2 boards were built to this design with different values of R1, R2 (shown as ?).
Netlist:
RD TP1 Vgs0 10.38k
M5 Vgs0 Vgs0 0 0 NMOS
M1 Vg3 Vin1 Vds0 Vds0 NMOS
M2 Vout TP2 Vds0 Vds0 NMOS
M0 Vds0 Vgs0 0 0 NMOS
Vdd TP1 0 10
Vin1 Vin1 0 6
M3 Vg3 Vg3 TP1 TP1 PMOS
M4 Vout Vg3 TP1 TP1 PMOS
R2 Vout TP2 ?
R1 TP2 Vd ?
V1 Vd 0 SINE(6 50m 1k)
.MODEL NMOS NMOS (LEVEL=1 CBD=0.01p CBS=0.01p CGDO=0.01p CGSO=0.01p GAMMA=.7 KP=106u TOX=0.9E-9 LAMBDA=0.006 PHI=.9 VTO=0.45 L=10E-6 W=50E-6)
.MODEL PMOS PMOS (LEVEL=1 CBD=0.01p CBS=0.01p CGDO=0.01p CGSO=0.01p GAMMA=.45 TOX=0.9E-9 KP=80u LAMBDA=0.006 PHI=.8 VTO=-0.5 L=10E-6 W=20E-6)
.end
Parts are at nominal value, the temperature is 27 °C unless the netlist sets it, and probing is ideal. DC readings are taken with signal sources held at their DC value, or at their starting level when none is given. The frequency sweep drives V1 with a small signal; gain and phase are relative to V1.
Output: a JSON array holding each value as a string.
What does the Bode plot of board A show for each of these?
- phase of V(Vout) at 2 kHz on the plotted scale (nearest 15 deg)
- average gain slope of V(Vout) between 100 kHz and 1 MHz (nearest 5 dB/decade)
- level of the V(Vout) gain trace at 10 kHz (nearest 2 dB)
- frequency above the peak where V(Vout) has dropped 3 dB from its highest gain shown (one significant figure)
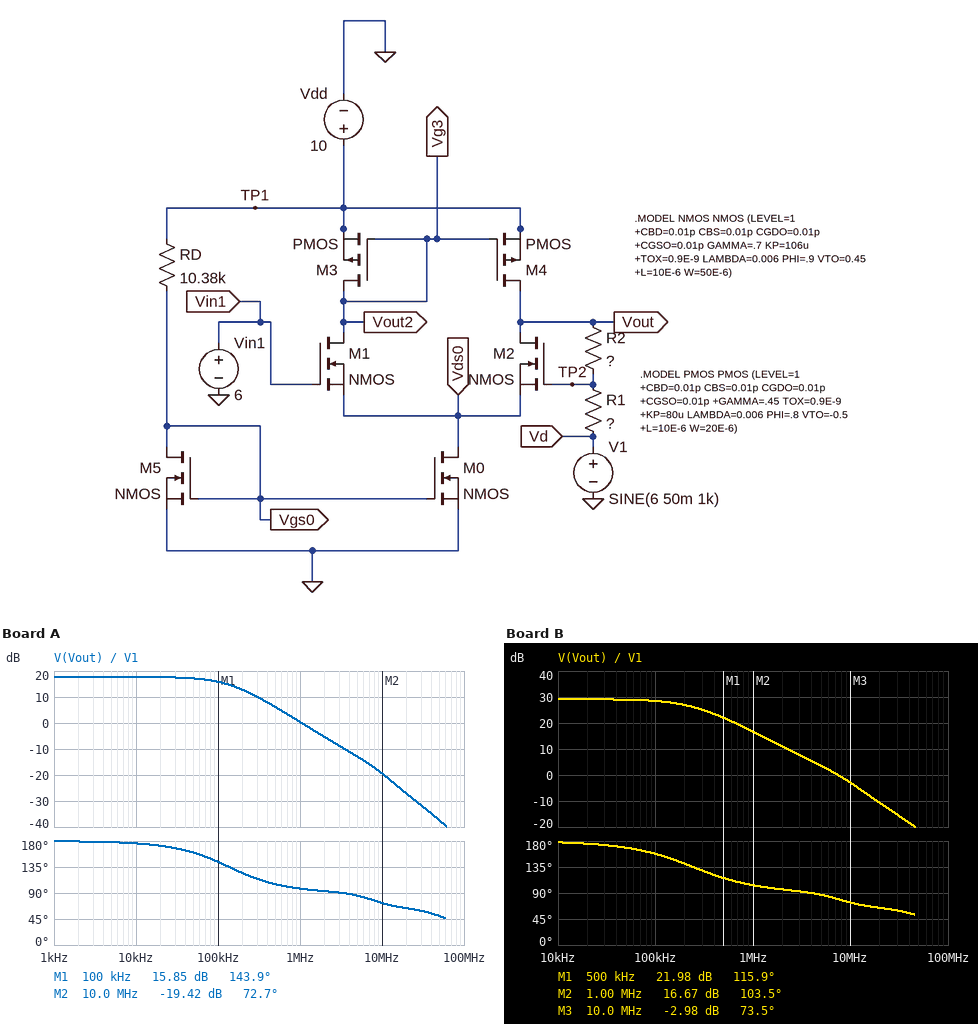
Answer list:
["180 deg", "-15 dB/decade", "18 dB", "100 kHz"]
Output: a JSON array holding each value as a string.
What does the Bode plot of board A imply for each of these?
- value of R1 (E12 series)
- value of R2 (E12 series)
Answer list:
["2.2 MΩ", "18 MΩ"]
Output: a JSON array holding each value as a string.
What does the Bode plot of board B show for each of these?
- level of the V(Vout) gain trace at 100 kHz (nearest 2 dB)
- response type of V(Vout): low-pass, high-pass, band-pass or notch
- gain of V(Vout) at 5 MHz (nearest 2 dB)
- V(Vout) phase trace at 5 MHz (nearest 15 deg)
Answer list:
["28 dB", "low-pass", "4 dB", "90 deg"]
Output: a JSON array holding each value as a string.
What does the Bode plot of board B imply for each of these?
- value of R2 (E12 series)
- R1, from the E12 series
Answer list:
["12 MΩ", "330 kΩ"]
